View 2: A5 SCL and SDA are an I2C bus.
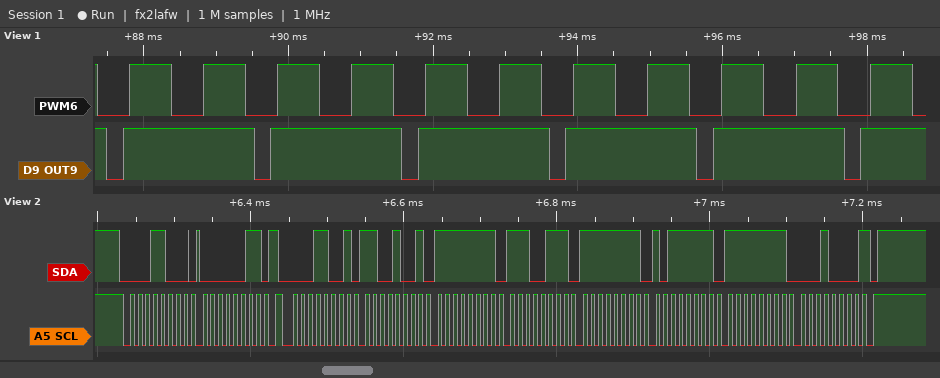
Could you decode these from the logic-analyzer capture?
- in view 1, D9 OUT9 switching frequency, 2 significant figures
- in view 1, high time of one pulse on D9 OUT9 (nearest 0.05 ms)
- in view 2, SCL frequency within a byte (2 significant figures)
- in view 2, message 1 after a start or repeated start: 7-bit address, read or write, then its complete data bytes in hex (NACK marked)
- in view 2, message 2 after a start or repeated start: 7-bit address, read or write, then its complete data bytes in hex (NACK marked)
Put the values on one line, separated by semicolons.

490 Hz; 1.80 ms; 100 kHz; 0x0C write: 03; 0x0C read: C9 FF E7 FF BF FF 10 NACK
